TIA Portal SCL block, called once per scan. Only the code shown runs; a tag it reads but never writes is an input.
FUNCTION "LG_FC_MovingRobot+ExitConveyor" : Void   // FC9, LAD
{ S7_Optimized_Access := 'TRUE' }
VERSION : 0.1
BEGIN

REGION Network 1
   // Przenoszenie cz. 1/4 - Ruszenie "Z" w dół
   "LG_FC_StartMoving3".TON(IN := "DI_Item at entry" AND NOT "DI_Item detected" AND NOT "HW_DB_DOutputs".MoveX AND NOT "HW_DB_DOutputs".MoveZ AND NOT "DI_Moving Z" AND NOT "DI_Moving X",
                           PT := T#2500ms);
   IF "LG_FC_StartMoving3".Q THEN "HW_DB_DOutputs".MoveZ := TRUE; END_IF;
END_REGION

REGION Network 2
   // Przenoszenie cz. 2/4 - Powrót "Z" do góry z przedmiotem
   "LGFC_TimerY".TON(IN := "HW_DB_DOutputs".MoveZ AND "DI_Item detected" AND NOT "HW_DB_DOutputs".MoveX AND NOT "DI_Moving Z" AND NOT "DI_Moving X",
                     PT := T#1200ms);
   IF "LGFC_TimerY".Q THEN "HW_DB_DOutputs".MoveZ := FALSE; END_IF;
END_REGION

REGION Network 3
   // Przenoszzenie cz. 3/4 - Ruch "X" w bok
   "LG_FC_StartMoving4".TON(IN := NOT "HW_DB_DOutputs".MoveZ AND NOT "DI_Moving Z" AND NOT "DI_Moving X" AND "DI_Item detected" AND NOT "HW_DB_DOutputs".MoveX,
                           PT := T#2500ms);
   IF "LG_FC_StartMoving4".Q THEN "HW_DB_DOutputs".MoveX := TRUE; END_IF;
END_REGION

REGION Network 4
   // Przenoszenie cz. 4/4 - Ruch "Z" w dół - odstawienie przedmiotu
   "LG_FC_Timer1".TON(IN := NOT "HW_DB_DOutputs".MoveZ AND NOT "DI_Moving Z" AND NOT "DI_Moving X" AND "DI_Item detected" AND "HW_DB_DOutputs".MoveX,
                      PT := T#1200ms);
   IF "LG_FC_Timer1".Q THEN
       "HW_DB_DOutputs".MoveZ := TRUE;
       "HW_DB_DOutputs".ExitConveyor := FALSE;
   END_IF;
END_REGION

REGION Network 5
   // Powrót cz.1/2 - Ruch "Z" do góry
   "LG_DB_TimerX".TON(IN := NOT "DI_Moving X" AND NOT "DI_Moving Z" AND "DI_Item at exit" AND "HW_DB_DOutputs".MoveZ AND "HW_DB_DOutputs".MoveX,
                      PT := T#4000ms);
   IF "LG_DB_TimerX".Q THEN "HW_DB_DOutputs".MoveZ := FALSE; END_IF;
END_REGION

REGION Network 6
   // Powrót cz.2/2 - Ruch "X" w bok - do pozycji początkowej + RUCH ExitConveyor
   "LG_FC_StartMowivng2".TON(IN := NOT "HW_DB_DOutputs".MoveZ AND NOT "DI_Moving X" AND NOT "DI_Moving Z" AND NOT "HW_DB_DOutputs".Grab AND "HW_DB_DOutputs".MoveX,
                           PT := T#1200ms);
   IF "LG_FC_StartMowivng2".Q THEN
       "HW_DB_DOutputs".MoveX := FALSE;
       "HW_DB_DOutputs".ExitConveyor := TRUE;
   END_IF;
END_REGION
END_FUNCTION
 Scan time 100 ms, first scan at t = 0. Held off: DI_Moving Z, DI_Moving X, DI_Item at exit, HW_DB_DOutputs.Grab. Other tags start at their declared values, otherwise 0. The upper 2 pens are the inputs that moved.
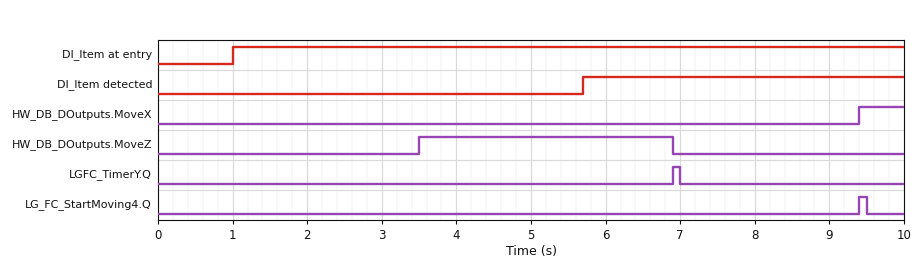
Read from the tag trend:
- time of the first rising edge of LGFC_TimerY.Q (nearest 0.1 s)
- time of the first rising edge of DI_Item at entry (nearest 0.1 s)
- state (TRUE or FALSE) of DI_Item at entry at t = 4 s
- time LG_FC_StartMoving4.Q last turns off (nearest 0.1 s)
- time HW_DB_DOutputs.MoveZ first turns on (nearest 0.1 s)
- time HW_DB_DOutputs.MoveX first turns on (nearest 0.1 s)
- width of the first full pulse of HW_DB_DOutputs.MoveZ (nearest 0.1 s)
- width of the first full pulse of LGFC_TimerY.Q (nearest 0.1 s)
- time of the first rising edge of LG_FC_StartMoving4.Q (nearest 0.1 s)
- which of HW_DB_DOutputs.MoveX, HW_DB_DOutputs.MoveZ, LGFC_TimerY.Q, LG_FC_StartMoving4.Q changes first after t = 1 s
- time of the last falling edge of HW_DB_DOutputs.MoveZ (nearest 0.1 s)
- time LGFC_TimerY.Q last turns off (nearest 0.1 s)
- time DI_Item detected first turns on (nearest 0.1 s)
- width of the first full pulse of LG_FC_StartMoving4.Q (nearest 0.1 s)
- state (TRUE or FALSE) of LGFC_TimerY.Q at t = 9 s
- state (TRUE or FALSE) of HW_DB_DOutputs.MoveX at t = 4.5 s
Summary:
6.9 s
1.0 s
TRUE
9.5 s
3.5 s
9.4 s
3.4 s
0.1 s
9.4 s
HW_DB_DOutputs.MoveZ
6.9 s
7.0 s
5.7 s
0.1 s
FALSE
FALSE
